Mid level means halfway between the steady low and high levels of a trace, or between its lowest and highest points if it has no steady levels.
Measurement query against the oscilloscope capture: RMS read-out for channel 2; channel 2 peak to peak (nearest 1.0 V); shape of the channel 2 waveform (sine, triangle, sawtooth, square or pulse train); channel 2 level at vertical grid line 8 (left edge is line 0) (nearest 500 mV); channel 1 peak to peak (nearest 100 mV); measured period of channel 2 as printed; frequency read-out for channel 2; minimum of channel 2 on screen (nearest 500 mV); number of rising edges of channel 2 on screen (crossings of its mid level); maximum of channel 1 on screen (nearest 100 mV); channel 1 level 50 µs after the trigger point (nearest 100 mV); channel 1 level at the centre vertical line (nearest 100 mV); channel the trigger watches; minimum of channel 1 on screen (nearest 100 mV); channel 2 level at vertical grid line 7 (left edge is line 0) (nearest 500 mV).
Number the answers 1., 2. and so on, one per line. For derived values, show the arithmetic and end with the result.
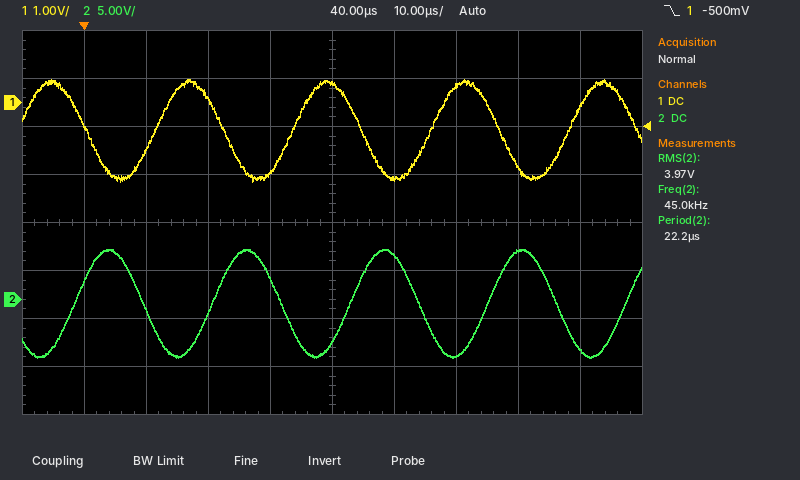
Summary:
1. 3.97 V
2. 11.0 V
3. sine
4. 5.0 V
5. 500 mV − (-1.6 V) = 2.1 V
6. 22.2 µs
7. 45.0 kHz
8. -6.0 V
9. 5
10. 500 mV
11. -1.6 V
12. 400 mV
13. channel 1
14. -1.6 V
15. -6.0 V
